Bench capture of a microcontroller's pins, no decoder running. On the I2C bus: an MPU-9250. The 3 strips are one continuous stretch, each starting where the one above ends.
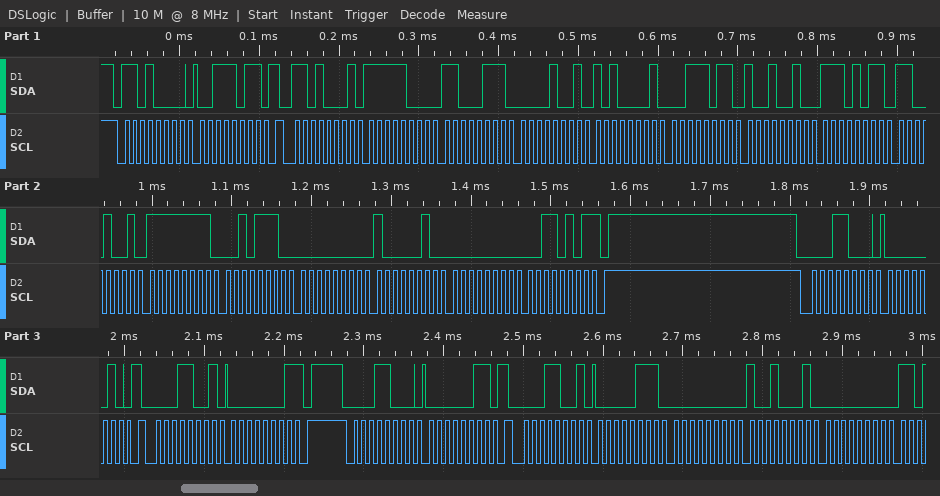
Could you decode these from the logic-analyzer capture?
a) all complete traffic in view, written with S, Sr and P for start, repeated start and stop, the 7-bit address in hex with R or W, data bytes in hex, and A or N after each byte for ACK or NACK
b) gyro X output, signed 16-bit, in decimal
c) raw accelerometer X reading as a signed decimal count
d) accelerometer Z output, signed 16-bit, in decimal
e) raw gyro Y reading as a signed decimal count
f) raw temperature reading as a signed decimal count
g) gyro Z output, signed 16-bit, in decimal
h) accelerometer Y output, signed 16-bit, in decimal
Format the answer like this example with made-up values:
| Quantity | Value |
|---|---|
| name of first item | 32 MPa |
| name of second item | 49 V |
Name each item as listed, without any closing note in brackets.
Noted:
| Quantity | Value |
|---|---|
| all complete traffic in view, written with S, Sr and P for start, repeated start and stop, the 7-bit address in hex with R or W, data bytes in hex, and A or N after each byte for ACK or NACK | S 68W A 3B A Sr 68R A F8 A C7 A 09 A A1 A 3B A 92 A EB A C9 A FF A 2E A 00 A 82 A 00 A 35 N P S 0CW A 02 A Sr 0CR A 01 N P S 0CW A 03 A Sr 0CR A 07 A 00 A 91 A 00 A |
| gyro X output, signed 16-bit, in decimal | -210 |
| raw accelerometer X reading as a signed decimal count | -1849 |
| accelerometer Z output, signed 16-bit, in decimal | 15250 |
| raw gyro Y reading as a signed decimal count | 130 |
| raw temperature reading as a signed decimal count | -5175 |
| gyro Z output, signed 16-bit, in decimal | 53 |
| accelerometer Y output, signed 16-bit, in decimal | 2465 |
